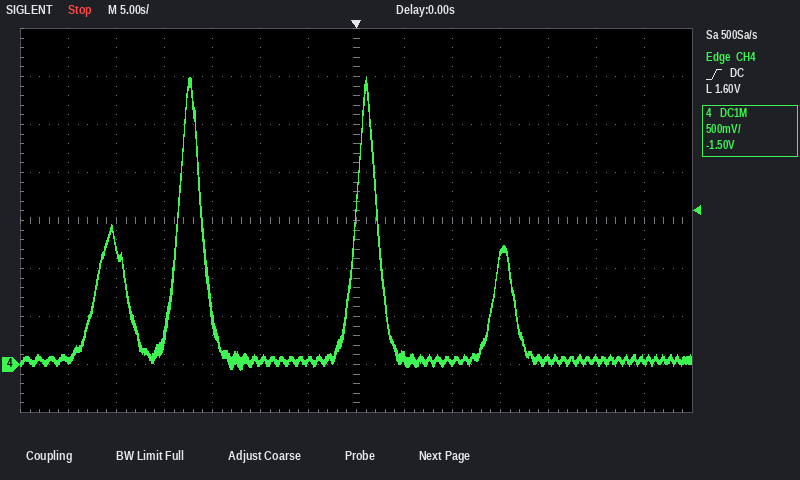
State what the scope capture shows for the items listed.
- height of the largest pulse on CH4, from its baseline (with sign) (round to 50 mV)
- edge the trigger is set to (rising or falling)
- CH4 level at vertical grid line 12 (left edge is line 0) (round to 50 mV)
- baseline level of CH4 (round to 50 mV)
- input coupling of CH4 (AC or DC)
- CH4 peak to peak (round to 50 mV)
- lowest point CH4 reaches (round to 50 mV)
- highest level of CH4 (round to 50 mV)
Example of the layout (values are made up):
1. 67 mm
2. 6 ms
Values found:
1. +2.95 V
2. rising
3. 50 mV
4. 50 mV
5. DC
6. 3.05 V
7. -50 mV
8. 3.00 V
